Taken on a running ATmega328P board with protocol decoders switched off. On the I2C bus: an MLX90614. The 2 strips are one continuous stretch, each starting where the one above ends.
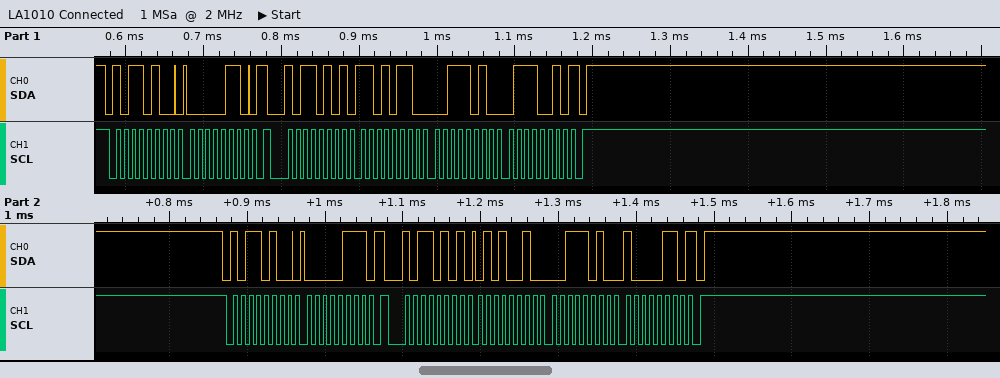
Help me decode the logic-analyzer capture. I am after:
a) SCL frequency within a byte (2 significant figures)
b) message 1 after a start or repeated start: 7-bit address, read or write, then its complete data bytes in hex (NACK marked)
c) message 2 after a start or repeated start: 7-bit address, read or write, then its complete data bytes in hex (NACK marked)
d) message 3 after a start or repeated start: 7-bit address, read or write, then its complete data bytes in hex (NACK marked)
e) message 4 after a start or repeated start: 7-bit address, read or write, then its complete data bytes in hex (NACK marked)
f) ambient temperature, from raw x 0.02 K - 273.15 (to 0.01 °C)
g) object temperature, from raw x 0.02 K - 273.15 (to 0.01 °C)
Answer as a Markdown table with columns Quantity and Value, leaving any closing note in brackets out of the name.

| Quantity | Value |
|---|---|
| SCL frequency within a byte | 100 kHz |
| message 1 after a start or repeated start: 7-bit address, read or write, then its complete data bytes in hex | 0x5A write: 06 |
| message 2 after a start or repeated start: 7-bit address, read or write, then its complete data bytes in hex | 0x5A read: D6 3A 72 NACK |
| message 3 after a start or repeated start: 7-bit address, read or write, then its complete data bytes in hex | 0x5A write: 07 |
| message 4 after a start or repeated start: 7-bit address, read or write, then its complete data bytes in hex | 0x5A read: 52 3A 86 NACK |
| ambient temperature, from raw x 0.02 K - 273.15 | 28.09 °C |
| object temperature, from raw x 0.02 K - 273.15 | 25.45 °C |
